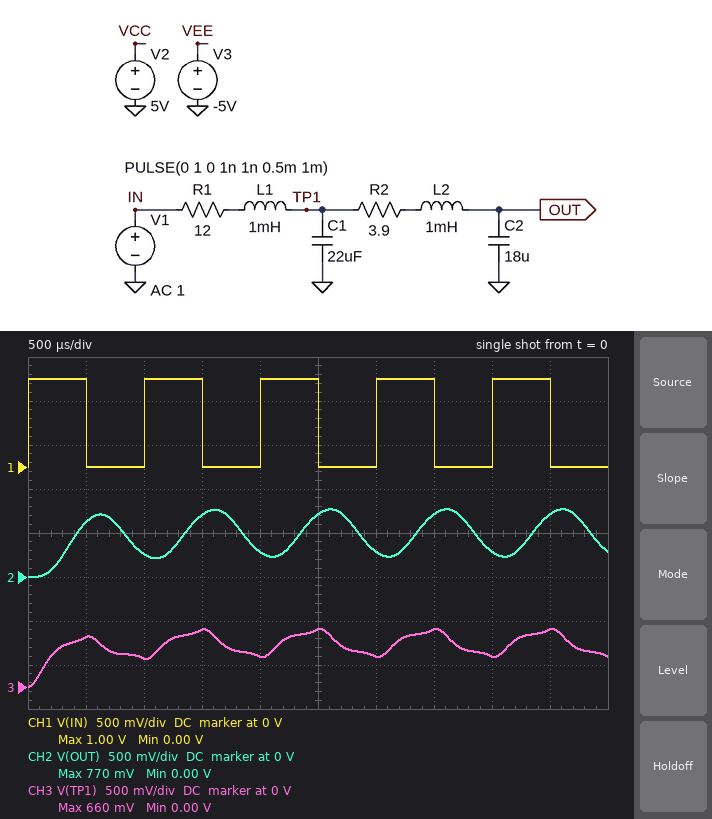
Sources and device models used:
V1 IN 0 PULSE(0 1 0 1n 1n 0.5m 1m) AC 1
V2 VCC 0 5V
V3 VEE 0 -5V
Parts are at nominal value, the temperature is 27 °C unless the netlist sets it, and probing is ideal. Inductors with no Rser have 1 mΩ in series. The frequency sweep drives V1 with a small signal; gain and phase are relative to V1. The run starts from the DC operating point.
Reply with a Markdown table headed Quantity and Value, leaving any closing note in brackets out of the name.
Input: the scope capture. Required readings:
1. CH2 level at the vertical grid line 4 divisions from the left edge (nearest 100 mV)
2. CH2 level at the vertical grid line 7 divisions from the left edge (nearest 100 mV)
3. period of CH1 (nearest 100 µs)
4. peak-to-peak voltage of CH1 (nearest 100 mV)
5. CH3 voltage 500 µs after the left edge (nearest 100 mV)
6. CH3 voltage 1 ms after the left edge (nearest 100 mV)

| Quantity | Value |
|---|---|
| CH2 level at the vertical grid line 4 divisions from the left edge | 300 mV |
| CH2 level at the vertical grid line 7 divisions from the left edge | 700 mV |
| period of CH1 | 1.0 ms |
| peak-to-peak voltage of CH1 | 1.0 V |
| CH3 voltage 500 µs after the left edge | 600 mV |
| CH3 voltage 1 ms after the left edge | 300 mV |
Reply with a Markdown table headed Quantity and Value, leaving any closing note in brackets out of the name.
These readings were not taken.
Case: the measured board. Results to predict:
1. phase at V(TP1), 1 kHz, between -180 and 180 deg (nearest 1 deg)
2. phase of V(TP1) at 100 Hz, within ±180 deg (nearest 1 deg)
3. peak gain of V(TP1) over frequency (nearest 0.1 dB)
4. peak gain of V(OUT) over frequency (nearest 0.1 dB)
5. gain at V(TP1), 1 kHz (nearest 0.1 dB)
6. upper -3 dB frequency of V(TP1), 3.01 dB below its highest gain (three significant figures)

| Quantity | Value |
|---|---|
| phase at V(TP1), 1 kHz, between -180 and 180 deg | -70 deg |
| phase of V(TP1) at 100 Hz, within ±180 deg | -17 deg |
| peak gain of V(TP1) over frequency | 0 dB |
| peak gain of V(OUT) over frequency | 0 dB |
| gain at V(TP1), 1 kHz | -13.0 dB |
| upper -3 dB frequency of V(TP1), 3.01 dB below its highest gain | 350 Hz |
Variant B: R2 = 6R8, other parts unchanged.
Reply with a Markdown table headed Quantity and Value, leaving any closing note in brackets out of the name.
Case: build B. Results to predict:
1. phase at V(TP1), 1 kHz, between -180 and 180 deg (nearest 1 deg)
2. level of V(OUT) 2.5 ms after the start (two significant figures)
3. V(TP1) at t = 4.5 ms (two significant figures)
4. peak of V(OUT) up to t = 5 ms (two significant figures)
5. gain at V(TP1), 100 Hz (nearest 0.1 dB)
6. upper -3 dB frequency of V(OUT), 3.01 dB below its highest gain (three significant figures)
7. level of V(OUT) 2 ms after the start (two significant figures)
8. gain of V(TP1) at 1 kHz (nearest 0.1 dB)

| Quantity | Value |
|---|---|
| phase at V(TP1), 1 kHz, between -180 and 180 deg | -66 deg |
| level of V(OUT) 2.5 ms after the start | 660 mV |
| V(TP1) at t = 4.5 ms | 700 mV |
| peak of V(OUT) up to t = 5 ms | 730 mV |
| gain at V(TP1), 100 Hz | -0.3 dB |
| upper -3 dB frequency of V(OUT), 3.01 dB below its highest gain | 373 Hz |
| level of V(OUT) 2 ms after the start | 340 mV |
| gain of V(TP1) at 1 kHz | -10.5 dB |
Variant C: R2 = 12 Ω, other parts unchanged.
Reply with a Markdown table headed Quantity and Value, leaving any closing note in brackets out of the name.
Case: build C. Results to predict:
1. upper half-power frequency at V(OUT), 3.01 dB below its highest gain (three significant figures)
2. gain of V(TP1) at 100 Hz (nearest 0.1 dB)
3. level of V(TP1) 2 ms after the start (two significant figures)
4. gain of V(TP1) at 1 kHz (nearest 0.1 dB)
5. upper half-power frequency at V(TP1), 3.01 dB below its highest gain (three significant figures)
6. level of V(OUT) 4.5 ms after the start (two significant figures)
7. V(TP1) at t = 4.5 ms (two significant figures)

| Quantity | Value |
|---|---|
| upper half-power frequency at V(OUT), 3.01 dB below its highest gain | 314 Hz |
| gain of V(TP1) at 100 Hz | -0.4 dB |
| level of V(TP1) 2 ms after the start | 240 mV |
| gain of V(TP1) at 1 kHz | -8.2 dB |
| upper half-power frequency at V(TP1), 3.01 dB below its highest gain | 329 Hz |
| level of V(OUT) 4.5 ms after the start | 600 mV |
| V(TP1) at t = 4.5 ms | 750 mV |
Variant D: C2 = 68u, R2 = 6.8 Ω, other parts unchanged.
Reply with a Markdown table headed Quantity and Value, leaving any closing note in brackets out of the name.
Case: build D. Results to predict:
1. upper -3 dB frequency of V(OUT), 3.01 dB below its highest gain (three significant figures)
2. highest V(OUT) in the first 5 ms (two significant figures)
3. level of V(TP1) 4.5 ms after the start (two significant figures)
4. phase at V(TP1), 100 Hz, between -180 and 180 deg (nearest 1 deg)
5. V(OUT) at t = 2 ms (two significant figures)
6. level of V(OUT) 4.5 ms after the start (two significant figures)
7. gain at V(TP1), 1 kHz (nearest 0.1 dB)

| Quantity | Value |
|---|---|
| upper -3 dB frequency of V(OUT), 3.01 dB below its highest gain | 118 Hz |
| highest V(OUT) in the first 5 ms | 560 mV |
| level of V(TP1) 4.5 ms after the start | 680 mV |
| phase at V(TP1), 100 Hz, between -180 and 180 deg | -31 deg |
| V(OUT) at t = 2 ms | 370 mV |
| level of V(OUT) 4.5 ms after the start | 510 mV |
| gain at V(TP1), 1 kHz | -7.7 dB |
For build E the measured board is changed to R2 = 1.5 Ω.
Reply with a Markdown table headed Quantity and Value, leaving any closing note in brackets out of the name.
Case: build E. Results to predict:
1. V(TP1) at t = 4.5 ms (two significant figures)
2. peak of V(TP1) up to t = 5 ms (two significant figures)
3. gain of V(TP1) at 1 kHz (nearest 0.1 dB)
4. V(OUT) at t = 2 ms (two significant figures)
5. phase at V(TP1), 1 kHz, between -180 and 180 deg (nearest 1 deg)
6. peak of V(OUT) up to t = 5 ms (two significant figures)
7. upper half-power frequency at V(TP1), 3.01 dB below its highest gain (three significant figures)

| Quantity | Value |
|---|---|
| V(TP1) at t = 4.5 ms | 620 mV |
| peak of V(TP1) up to t = 5 ms | 640 mV |
| gain of V(TP1) at 1 kHz | -15.9 dB |
| V(OUT) at t = 2 ms | 230 mV |
| phase at V(TP1), 1 kHz, between -180 and 180 deg | -87 deg |
| peak of V(OUT) up to t = 5 ms | 800 mV |
| upper half-power frequency at V(TP1), 3.01 dB below its highest gain | 364 Hz |
